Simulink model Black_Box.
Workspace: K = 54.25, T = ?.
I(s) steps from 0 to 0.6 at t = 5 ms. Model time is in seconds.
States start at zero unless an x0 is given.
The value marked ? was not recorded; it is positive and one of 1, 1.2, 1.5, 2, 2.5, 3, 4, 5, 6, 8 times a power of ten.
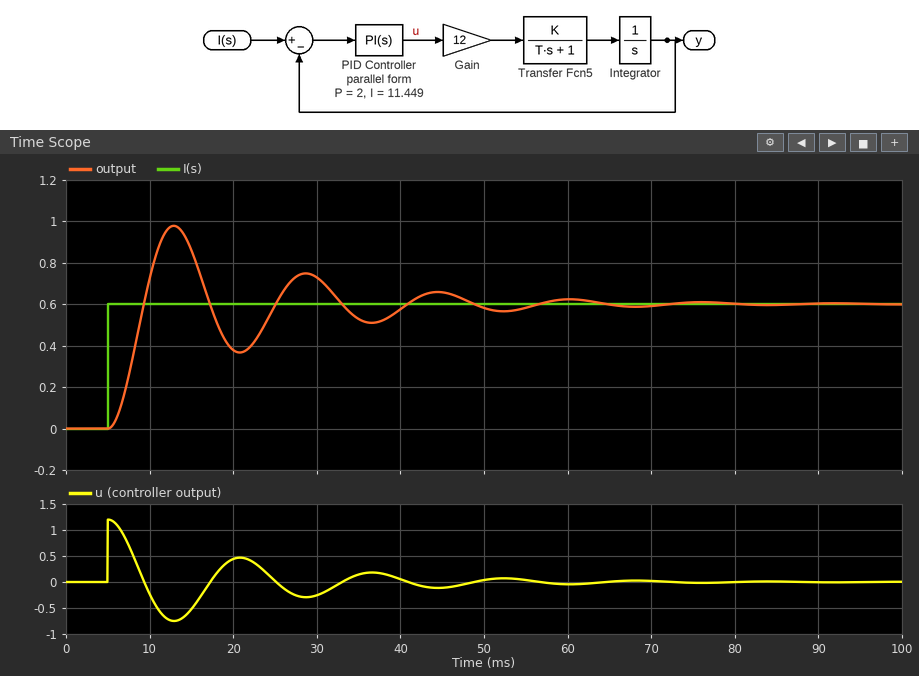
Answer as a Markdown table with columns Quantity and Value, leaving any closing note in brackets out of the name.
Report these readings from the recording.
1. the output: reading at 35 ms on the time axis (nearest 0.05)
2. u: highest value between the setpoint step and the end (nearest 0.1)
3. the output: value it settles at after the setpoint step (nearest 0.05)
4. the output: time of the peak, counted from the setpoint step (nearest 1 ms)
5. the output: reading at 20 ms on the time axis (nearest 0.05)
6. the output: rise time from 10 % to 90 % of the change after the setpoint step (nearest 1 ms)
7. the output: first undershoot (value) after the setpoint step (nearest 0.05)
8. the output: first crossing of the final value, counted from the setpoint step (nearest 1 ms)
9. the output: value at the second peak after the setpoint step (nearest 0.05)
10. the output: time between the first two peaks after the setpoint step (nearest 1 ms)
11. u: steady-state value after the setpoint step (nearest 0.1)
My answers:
| Quantity | Value |
|---|---|
| the output: reading at 35 ms on the time axis | 0.55 |
| u: highest value between the setpoint step and the end | 1.2 |
| the output: value it settles at after the setpoint step | 0.60 |
| the output: time of the peak, counted from the setpoint step | 8 ms |
| the output: reading at 20 ms on the time axis | 0.40 |
| the output: rise time from 10 % to 90 % of the change after the setpoint step | 3 ms |
| the output: first undershoot (value) after the setpoint step | 0.35 |
| the output: first crossing of the final value, counted from the setpoint step | 4 ms |
| the output: value at the second peak after the setpoint step | 0.75 |
| the output: time between the first two peaks after the setpoint step | 16 ms |
| u: steady-state value after the setpoint step | 0.0 |
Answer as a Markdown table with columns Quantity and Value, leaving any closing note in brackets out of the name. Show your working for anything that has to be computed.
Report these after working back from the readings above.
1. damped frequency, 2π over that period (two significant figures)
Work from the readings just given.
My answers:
| Quantity | Value |
|---|---|
| damped frequency, 2π over that period | 2π / 16 = 0.39 rad/ms |
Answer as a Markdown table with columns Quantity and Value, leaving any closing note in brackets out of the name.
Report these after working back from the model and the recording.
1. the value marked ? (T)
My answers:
| Quantity | Value |
|---|---|
| the value marked ? | 0.008 |
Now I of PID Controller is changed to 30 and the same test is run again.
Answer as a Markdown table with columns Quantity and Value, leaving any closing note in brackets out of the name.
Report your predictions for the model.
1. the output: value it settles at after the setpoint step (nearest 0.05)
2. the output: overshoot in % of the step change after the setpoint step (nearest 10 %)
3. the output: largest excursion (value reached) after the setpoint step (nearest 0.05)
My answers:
| Quantity | Value |
|---|---|
| the output: value it settles at after the setpoint step | 0.60 |
| the output: overshoot in % of the step change after the setpoint step | 70 % |
| the output: largest excursion (value reached) after the setpoint step | 1.00 |
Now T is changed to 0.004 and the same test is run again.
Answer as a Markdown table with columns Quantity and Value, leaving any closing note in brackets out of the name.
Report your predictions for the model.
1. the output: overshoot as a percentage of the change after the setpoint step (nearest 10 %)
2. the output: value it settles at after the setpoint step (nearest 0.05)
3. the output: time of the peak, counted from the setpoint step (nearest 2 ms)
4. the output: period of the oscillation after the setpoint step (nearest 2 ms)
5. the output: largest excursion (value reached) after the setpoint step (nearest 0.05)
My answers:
| Quantity | Value |
|---|---|
| the output: overshoot as a percentage of the change after the setpoint step | 50 % |
| the output: value it settles at after the setpoint step | 0.60 |
| the output: time of the peak, counted from the setpoint step | 6 ms |
| the output: period of the oscillation after the setpoint step | 12 ms |
| the output: largest excursion (value reached) after the setpoint step | 0.90 |
